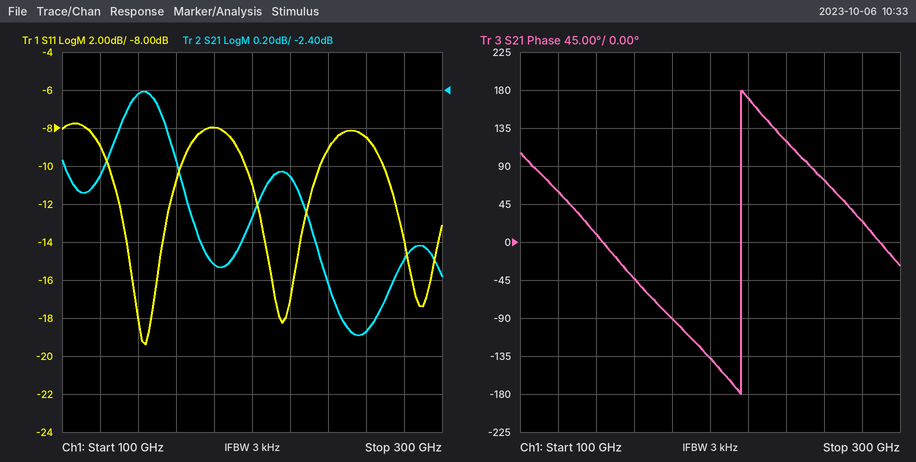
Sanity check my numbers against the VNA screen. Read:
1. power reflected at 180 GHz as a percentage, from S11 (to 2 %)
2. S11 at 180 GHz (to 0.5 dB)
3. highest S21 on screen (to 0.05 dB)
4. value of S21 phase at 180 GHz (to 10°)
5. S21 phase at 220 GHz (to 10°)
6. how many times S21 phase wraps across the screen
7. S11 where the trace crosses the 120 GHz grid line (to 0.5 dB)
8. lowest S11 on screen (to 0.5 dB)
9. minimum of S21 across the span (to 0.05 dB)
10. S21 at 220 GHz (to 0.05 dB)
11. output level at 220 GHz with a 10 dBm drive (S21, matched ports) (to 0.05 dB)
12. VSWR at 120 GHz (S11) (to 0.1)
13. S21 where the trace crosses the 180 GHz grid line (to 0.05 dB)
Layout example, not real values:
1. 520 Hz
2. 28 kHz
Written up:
1. 16 %
2. -8.0 dB
3. -2.40 dB
4. -90°
5. 170°
6. 1
7. -9.0 dB
8. -19.5 dB
9. -3.70 dB
10. -2.85 dB
11. 7.15 dBm
12. 2.1
13. -3.30 dB
